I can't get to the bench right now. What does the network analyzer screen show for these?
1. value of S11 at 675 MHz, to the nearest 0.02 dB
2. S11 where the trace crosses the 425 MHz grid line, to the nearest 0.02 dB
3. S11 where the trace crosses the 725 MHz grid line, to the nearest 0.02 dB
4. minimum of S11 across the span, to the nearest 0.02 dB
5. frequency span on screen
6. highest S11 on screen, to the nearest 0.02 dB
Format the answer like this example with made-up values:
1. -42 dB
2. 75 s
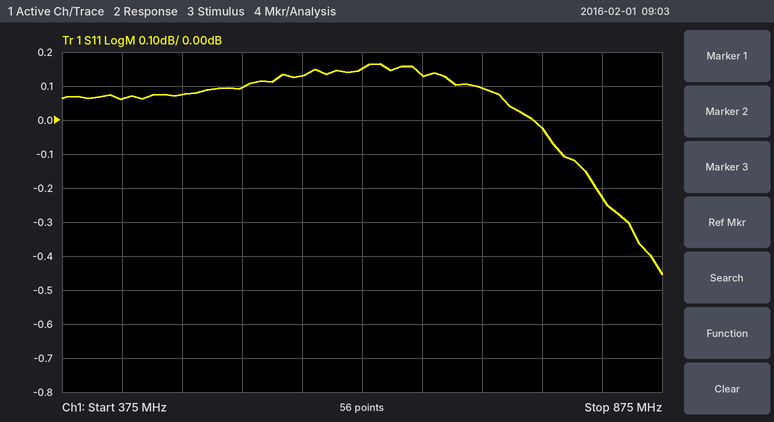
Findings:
1. 0.14 dB
2. 0.06 dB
3. 0.10 dB
4. -0.46 dB
5. 500 MHz
6. 0.16 dB
